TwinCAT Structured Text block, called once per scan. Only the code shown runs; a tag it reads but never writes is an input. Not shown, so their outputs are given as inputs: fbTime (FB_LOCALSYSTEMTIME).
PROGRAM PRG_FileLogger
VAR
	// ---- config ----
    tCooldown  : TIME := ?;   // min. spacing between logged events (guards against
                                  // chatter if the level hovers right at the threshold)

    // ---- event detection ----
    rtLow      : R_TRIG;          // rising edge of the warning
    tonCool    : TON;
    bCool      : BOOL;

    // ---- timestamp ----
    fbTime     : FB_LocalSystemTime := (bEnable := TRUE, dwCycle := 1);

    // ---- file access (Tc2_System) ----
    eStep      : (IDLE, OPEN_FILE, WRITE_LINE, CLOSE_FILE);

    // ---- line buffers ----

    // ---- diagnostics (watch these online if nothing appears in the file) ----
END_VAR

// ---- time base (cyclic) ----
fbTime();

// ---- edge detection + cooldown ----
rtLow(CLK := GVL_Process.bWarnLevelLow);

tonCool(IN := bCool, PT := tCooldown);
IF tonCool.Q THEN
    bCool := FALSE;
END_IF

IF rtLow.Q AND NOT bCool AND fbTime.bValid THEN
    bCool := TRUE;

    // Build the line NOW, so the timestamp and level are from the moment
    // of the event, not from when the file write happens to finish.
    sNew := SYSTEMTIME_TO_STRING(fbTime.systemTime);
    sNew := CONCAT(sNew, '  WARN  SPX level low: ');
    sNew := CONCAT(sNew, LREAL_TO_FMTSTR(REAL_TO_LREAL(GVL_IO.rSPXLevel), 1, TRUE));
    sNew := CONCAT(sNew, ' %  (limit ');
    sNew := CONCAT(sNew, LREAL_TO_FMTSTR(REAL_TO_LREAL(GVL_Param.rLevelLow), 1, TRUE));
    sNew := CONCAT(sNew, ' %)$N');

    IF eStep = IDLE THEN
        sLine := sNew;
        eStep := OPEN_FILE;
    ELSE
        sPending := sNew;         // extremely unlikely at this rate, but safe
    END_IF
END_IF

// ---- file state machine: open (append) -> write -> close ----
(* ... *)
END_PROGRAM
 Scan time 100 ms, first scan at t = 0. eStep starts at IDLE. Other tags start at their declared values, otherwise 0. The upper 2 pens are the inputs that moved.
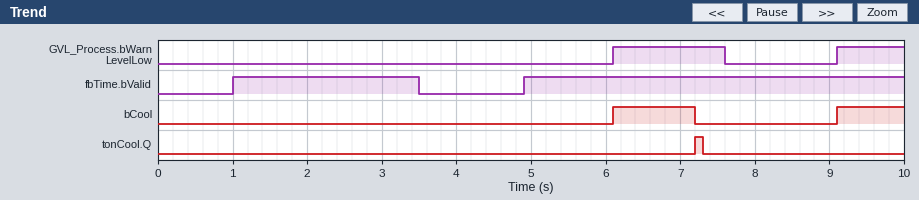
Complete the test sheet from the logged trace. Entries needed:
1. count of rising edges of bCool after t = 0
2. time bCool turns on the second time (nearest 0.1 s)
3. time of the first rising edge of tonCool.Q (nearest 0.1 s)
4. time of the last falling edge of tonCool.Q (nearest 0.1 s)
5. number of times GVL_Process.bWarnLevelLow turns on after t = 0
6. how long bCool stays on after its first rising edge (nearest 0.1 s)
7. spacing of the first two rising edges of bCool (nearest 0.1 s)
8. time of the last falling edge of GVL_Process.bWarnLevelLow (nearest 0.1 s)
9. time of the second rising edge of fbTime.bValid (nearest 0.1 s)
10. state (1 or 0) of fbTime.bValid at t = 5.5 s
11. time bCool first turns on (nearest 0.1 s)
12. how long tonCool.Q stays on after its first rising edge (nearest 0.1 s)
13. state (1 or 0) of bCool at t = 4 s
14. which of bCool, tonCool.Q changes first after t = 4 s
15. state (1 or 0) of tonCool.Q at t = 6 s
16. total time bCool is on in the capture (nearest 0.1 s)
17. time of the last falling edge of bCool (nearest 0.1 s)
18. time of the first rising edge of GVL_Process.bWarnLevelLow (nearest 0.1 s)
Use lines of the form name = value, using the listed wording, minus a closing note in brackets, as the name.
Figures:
count of rising edges of bCool after t = 0 = 2
time bCool turns on the second time = 9.1 s
time of the first rising edge of tonCool.Q = 7.2 s
time of the last falling edge of tonCool.Q = 7.3 s
number of times GVL_Process.bWarnLevelLow turns on after t = 0 = 2
how long bCool stays on after its first rising edge = 1.1 s
spacing of the first two rising edges of bCool = 3.0 s
time of the last falling edge of GVL_Process.bWarnLevelLow = 7.6 s
time of the second rising edge of fbTime.bValid = 4.9 s
state (1 or 0) of fbTime.bValid at t = 5.5 s = 1
time bCool first turns on = 6.1 s
how long tonCool.Q stays on after its first rising edge = 0.1 s
state (1 or 0) of bCool at t = 4 s = 0
which of bCool, tonCool.Q changes first after t = 4 s = bCool
state (1 or 0) of tonCool.Q at t = 6 s = 0
total time bCool is on in the capture = 2.0 s
time of the last falling edge of bCool = 7.2 s
time of the first rising edge of GVL_Process.bWarnLevelLow = 6.1 s
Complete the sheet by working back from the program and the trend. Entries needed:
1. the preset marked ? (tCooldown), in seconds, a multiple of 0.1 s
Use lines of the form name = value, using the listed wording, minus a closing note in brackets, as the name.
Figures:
the preset marked ? (tCooldown), in seconds, a multiple of 0.1 s = 1.0 s
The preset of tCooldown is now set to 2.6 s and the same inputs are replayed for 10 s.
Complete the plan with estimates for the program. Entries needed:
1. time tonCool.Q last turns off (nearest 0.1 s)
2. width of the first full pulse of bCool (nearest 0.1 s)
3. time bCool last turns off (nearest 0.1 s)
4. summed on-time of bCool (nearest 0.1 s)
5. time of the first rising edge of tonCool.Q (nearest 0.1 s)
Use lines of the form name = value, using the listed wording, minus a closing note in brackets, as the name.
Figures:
time tonCool.Q last turns off = 8.9 s
width of the first full pulse of bCool = 2.7 s
time bCool last turns off = 8.8 s
summed on-time of bCool = 3.6 s
time of the first rising edge of tonCool.Q = 8.8 s
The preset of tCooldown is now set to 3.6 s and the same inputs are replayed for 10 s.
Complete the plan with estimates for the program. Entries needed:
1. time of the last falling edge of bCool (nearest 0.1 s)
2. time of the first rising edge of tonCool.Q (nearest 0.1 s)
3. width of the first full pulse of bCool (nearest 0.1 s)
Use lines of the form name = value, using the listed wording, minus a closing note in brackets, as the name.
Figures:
time of the last falling edge of bCool = 9.8 s
time of the first rising edge of tonCool.Q = 9.8 s
width of the first full pulse of bCool = 3.7 s
